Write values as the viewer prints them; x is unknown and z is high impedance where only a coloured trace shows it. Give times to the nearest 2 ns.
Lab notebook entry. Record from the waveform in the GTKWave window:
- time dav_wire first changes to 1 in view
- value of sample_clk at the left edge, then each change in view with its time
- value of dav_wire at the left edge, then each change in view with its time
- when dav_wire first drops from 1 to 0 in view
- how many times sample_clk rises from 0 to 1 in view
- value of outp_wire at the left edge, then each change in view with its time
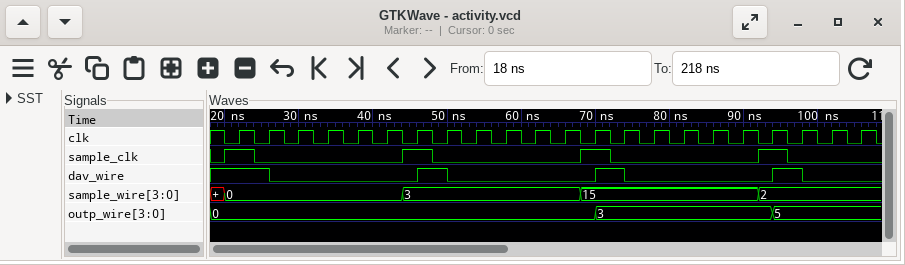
46 ns
0, 1 at 20 ns, 0 at 24 ns, 1 at 44 ns, 0 at 48 ns, 1 at 68 ns, 0 at 72 ns, 1 at 92 ns, 0 at 96 ns
1, 0 at 26 ns, 1 at 46 ns, 0 at 50 ns, 1 at 70 ns, 0 at 74 ns, 1 at 94 ns, 0 at 98 ns
26 ns
4
0, 3 at 70 ns, 5 at 94 ns
